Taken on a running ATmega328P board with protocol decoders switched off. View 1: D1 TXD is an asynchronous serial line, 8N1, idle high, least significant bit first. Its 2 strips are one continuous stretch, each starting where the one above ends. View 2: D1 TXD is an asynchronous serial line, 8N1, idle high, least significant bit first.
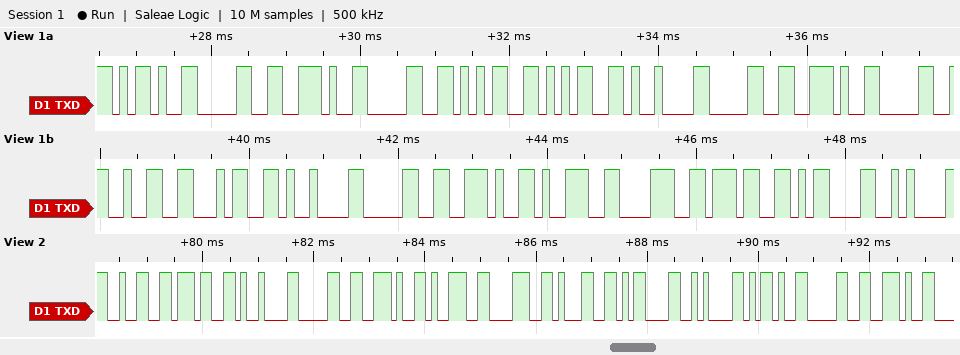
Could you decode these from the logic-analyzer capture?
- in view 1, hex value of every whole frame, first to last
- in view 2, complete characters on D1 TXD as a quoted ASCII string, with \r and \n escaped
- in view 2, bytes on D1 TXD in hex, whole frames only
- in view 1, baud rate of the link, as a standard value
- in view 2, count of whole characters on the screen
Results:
0x2D 0x30 0x2E 0x30 0x35 0x35 0x09 0x30 0x2E 0x30 0x32 0x34 0x09 0x30 0x2E 0x39 0x38 0x37 0x0D 0x0A
"27\t0.981\r\n-0."
32 37 09 30 2E 39 38 31 0D 0A 2D 30 2E
9600 baud
13
